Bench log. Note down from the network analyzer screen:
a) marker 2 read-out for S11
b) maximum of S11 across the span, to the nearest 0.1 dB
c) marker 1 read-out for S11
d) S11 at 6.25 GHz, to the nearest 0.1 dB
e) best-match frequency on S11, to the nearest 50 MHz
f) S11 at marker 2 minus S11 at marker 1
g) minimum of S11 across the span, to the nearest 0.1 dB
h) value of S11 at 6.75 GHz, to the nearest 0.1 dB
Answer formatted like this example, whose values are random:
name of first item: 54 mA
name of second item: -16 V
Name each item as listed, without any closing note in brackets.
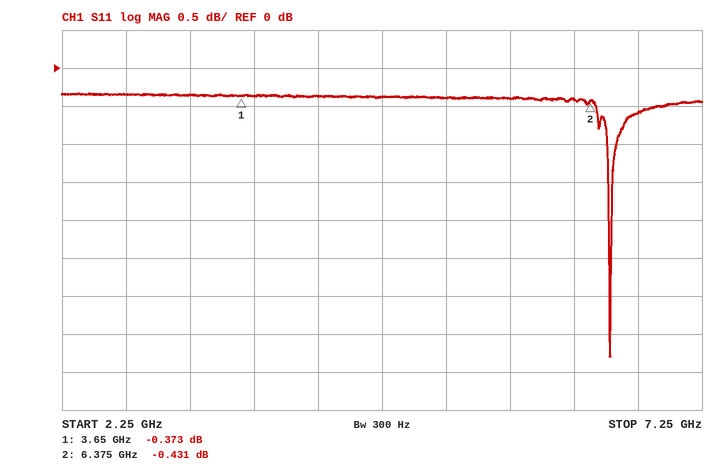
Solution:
marker 2 read-out for S11: -0.431 dB
maximum of S11 across the span, to the nearest 0.1 dB: -0.3 dB
marker 1 read-out for S11: -0.373 dB
S11 at 6.25 GHz, to the nearest 0.1 dB: -0.4 dB
best-match frequency on S11, to the nearest 50 MHz: 6.55 GHz
S11 at marker 2 minus S11 at marker 1: -0.058 dB
minimum of S11 across the span, to the nearest 0.1 dB: -3.8 dB
value of S11 at 6.75 GHz, to the nearest 0.1 dB: -0.6 dB
